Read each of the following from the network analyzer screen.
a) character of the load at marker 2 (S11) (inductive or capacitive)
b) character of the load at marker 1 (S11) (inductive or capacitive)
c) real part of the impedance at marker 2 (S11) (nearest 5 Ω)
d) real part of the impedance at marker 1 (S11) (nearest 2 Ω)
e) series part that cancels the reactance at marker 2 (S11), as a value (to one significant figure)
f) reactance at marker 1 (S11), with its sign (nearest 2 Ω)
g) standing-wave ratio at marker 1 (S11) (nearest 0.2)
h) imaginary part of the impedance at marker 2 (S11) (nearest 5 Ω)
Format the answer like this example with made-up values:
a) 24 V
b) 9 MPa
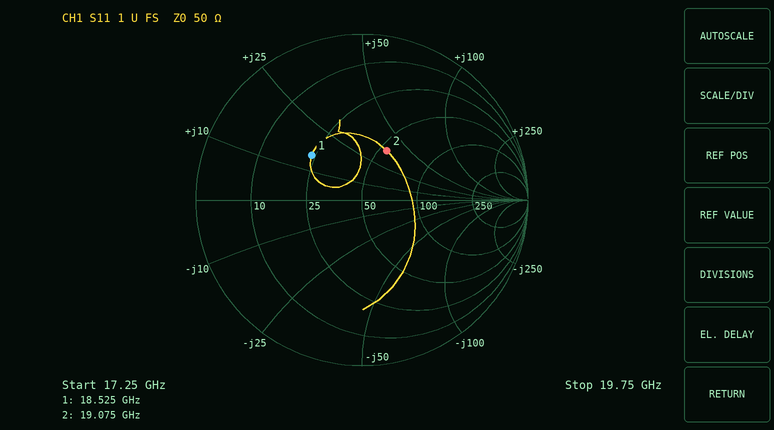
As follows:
a) inductive
b) inductive
c) 55 Ω
d) 24 Ω
e) 200 fF
f) +16 Ω
g) 2.4
h) +35 Ω
